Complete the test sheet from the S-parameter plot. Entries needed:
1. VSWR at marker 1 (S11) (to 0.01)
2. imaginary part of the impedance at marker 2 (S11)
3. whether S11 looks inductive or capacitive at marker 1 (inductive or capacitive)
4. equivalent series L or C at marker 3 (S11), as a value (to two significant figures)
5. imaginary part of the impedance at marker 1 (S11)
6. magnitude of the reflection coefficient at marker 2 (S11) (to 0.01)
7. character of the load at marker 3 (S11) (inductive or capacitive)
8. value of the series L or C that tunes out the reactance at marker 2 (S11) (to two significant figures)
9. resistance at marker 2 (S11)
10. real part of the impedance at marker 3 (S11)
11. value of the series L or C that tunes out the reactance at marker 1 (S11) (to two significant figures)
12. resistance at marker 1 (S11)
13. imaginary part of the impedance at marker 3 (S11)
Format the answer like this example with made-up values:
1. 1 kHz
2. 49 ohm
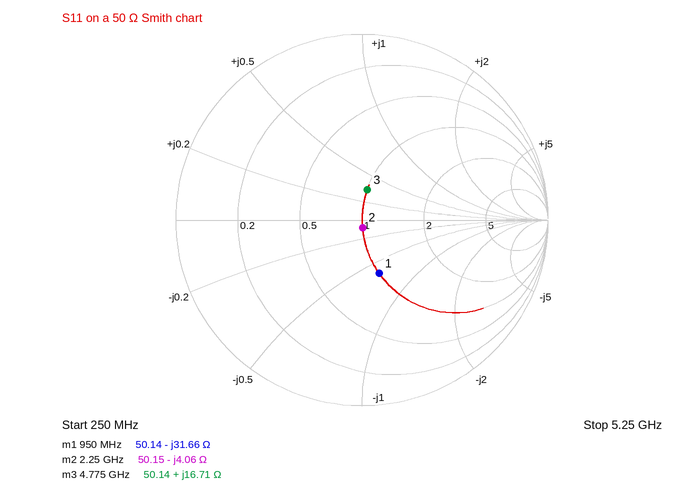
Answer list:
1. 1.86
2. -4.06 Ω
3. capacitive
4. 560 pH
5. -31.66 Ω
6. 0.04
7. inductive
8. 290 pH
9. 50.15 Ω
10. 50.14 Ω
11. 5.3 nH
12. 50.14 Ω
13. +16.71 Ω
